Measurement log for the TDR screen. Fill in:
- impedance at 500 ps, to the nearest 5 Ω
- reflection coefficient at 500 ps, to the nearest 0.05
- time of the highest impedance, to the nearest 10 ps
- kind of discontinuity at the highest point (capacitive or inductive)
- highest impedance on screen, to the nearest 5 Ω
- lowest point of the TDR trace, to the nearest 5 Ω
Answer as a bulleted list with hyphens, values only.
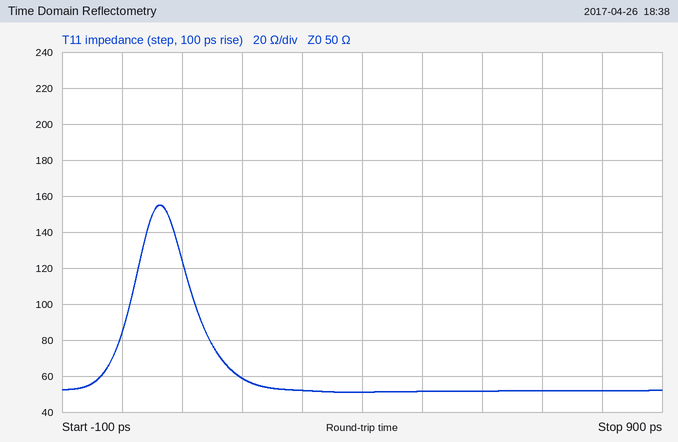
- 50 Ω
- 0.00
- 60 ps
- inductive
- 155 Ω
- 50 Ω
